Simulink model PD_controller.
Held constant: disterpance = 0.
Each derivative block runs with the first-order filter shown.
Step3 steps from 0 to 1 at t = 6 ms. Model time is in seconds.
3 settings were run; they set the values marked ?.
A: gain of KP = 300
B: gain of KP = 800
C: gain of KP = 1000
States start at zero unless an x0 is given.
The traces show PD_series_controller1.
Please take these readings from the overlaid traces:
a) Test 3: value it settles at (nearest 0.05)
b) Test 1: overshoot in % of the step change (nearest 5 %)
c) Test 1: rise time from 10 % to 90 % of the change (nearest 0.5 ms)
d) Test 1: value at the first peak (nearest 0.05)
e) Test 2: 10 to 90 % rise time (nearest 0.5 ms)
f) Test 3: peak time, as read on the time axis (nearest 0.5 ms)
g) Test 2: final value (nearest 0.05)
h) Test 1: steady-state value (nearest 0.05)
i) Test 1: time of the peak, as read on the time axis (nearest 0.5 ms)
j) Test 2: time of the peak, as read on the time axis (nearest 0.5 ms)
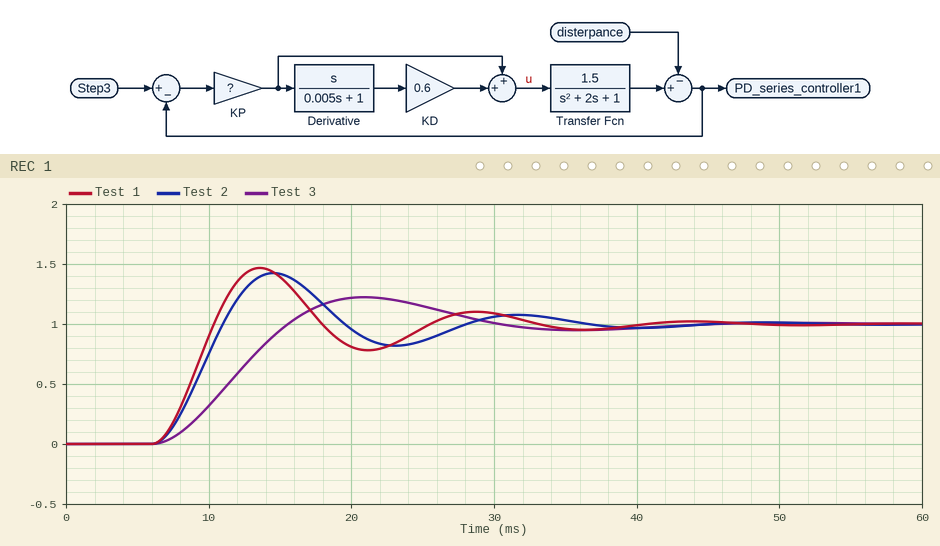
1.00
45 %
3.0 ms
1.45
3.5 ms
21.0 ms
1.00
1.00
13.5 ms
14.5 ms
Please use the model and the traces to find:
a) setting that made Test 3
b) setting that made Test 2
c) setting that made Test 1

A
B
C
